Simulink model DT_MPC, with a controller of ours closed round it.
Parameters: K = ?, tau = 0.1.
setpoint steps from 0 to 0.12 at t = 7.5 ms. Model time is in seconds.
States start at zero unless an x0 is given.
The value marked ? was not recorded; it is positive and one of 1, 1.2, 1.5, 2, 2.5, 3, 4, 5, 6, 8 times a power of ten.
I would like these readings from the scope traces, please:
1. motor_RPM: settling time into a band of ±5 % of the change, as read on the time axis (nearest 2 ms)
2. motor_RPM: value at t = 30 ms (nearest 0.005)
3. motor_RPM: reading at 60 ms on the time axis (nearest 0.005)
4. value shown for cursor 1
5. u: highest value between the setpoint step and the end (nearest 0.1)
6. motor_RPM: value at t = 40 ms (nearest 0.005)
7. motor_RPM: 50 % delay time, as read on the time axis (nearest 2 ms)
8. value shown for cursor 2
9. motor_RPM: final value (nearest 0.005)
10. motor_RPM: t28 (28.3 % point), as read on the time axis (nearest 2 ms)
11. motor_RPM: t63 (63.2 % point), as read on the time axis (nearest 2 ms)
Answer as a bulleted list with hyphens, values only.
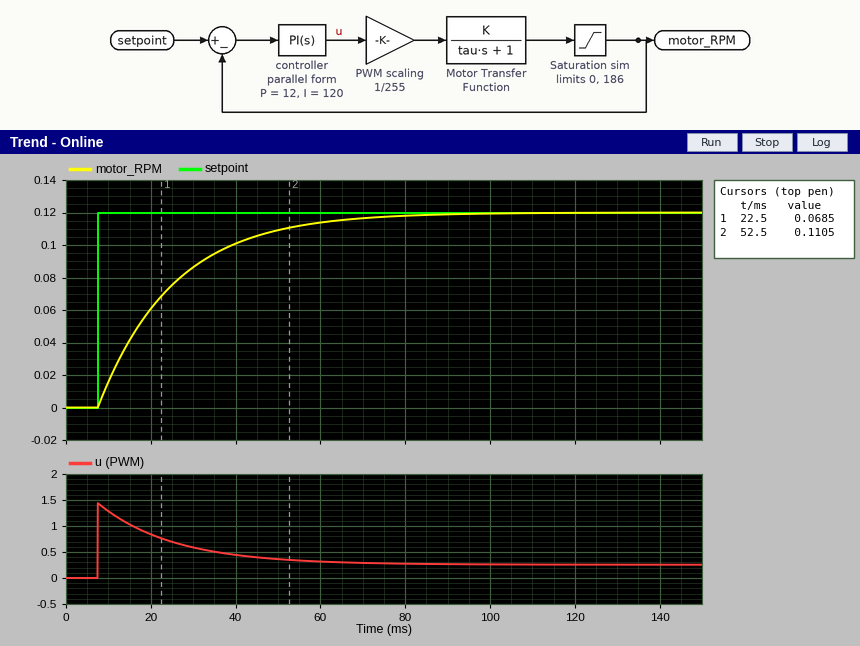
- 60 ms
- 0.085
- 0.115
- 0.0685
- 1.4
- 0.100
- 20 ms
- 0.1105
- 0.120
- 14 ms
- 26 ms
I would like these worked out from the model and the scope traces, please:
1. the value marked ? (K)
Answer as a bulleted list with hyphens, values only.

- 120
